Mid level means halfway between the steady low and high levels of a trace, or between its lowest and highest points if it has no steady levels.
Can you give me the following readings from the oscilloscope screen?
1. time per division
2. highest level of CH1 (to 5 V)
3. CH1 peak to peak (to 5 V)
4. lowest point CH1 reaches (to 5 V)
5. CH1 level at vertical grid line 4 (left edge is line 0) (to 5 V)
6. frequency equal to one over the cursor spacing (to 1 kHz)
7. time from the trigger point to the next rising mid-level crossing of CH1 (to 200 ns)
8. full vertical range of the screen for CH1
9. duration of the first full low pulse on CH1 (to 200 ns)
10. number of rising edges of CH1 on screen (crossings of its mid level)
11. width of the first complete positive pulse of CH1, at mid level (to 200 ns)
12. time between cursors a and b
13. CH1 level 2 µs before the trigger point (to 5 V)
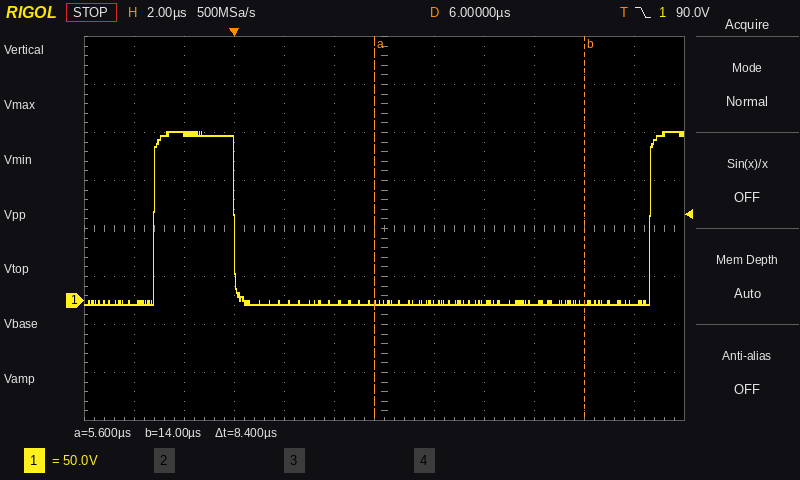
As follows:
2 µs
175 V
180 V
-5 V
-5 V
119 kHz
16.6 µs
400 V
16.6 µs
2
3.2 µs
8.4 µs
175 V
